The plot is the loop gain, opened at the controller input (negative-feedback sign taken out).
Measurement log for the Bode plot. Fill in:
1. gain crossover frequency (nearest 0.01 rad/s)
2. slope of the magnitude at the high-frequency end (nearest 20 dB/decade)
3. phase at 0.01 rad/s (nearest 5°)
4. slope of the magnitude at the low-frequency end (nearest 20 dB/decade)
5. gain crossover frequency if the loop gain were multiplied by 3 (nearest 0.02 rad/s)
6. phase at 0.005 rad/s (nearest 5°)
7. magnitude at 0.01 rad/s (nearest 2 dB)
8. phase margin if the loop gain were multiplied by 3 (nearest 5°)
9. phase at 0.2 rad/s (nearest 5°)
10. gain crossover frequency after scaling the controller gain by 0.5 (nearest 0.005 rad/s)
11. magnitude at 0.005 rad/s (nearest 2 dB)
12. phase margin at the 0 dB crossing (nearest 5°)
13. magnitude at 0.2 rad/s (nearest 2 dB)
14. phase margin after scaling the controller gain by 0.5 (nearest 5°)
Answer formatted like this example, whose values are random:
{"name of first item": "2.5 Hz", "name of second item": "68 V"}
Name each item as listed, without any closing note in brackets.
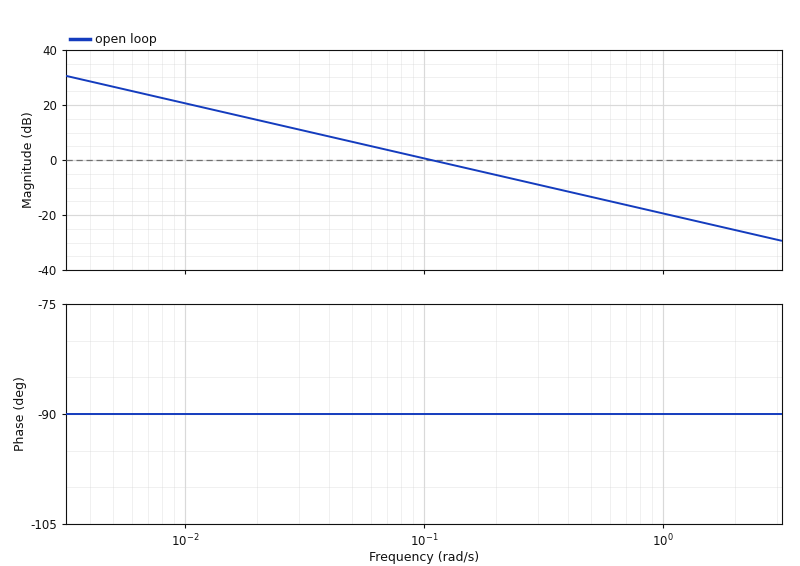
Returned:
{"gain crossover frequency": "0.11 rad/s", "slope of the magnitude at the high-frequency end": "-20 dB/decade", "phase at 0.01 rad/s": "-90°", "slope of the magnitude at the low-frequency end": "-20 dB/decade", "gain crossover frequency if the loop gain were multiplied by 3": "0.32 rad/s", "phase at 0.005 rad/s": "-90°", "magnitude at 0.01 rad/s": "20 dB", "phase margin if the loop gain were multiplied by 3": "90°", "phase at 0.2 rad/s": "-90°", "gain crossover frequency after scaling the controller gain by 0.5": "0.055 rad/s", "magnitude at 0.005 rad/s": "26 dB", "phase margin at the 0 dB crossing": "90°", "magnitude at 0.2 rad/s": "-6 dB", "phase margin after scaling the controller gain by 0.5": "90°"}
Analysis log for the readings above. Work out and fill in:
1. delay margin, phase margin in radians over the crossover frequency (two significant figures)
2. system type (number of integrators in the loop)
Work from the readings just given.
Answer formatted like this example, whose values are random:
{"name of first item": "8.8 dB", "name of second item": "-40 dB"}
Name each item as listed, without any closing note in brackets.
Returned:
{"delay margin, phase margin in radians over the crossover frequency": "14 s", "system type": "1"}
